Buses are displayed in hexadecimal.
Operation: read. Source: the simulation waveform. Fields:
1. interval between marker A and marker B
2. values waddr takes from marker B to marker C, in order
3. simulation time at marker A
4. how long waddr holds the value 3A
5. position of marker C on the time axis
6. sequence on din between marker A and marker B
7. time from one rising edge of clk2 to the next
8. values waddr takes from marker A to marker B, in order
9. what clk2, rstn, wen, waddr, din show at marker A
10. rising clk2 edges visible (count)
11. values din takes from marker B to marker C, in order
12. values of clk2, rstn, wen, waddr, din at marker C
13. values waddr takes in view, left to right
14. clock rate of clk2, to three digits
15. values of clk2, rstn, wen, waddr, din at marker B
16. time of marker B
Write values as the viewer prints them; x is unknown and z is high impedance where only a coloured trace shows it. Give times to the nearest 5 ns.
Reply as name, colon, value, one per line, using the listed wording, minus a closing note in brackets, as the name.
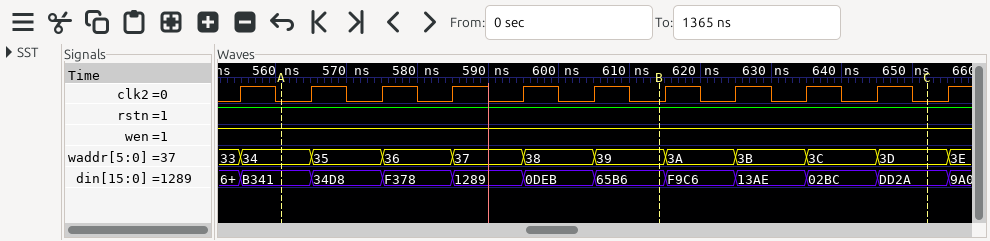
interval between marker A and marker B: 55 ns
values waddr takes from marker B to marker C, in order: 39, 3A, 3B, 3C, 3D
simulation time at marker A: 560 ns
how long waddr holds the value 3A: 10 ns
position of marker C on the time axis: 650 ns
sequence on din between marker A and marker B: B341, 34D8, F378, 1289, 0DEB, 65B6
time from one rising edge of clk2 to the next: 10 ns
values waddr takes from marker A to marker B, in order: 34, 35, 36, 37, 38, 39
what clk2, rstn, wen, waddr, din show at marker A: clk2=0, rstn=1, wen=1, waddr=34, din=B341
rising clk2 edges visible: 11
values din takes from marker B to marker C, in order: 65B6, F9C6, 13AE, 02BC, DD2A
values of clk2, rstn, wen, waddr, din at marker C: clk2=0, rstn=1, wen=1, waddr=3D, din=DD2A
values waddr takes in view, left to right: 33, 34, 35, 36, 37, 38, 39, 3A, 3B, 3C, 3D, 3E
clock rate of clk2, to three digits: 100 MHz
values of clk2, rstn, wen, waddr, din at marker B: clk2=0, rstn=1, wen=1, waddr=39, din=65B6
time of marker B: 615 ns
